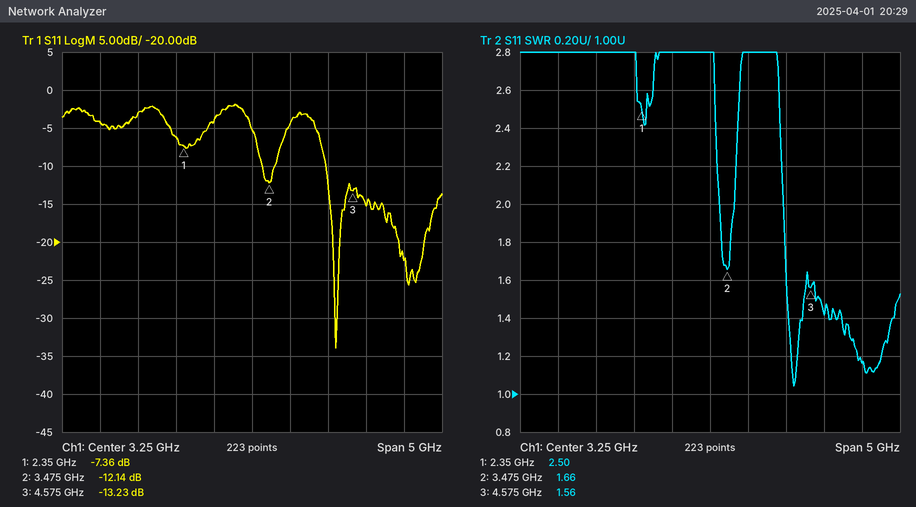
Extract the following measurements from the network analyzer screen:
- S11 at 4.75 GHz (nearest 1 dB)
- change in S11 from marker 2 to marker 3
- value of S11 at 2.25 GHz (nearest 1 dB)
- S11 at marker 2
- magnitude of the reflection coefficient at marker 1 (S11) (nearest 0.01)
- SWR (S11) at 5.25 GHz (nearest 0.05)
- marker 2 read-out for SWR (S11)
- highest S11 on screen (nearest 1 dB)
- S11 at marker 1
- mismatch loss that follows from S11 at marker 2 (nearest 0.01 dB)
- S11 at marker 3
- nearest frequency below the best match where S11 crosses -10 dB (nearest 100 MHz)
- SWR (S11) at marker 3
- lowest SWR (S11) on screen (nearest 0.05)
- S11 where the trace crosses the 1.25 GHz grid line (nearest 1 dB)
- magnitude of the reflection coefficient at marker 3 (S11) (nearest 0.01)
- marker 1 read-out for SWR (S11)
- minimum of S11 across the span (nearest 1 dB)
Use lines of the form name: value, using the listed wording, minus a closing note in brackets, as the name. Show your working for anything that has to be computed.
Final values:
S11 at 4.75 GHz: -15 dB
change in S11 from marker 2 to marker 3: -13.23 − (-12.14) = -1.09 dB
value of S11 at 2.25 GHz: -6 dB
S11 at marker 2: -12.14 dB
magnitude of the reflection coefficient at marker 1 (S11): 10^(-7.36/20) ≈ 0.43
SWR (S11) at 5.25 GHz: 1.15
marker 2 read-out for SWR: 1.66
highest S11 on screen: -2 dB
S11 at marker 1: -7.36 dB
mismatch loss that follows from S11 at marker 2: −10 log10(1 − 10^(-12.14/10)) ≈ 0.27 dB
S11 at marker 3: -13.23 dB
nearest frequency below the best match where S11 crosses -10 dB: 4.2 GHz
SWR (S11) at marker 3: 1.56
lowest SWR (S11) on screen: 1.05
S11 where the trace crosses the 1.25 GHz grid line: -4 dB
magnitude of the reflection coefficient at marker 3 (S11): 10^(-13.23/20) ≈ 0.22
marker 1 read-out for SWR: 2.50
minimum of S11 across the span: -34 dB
